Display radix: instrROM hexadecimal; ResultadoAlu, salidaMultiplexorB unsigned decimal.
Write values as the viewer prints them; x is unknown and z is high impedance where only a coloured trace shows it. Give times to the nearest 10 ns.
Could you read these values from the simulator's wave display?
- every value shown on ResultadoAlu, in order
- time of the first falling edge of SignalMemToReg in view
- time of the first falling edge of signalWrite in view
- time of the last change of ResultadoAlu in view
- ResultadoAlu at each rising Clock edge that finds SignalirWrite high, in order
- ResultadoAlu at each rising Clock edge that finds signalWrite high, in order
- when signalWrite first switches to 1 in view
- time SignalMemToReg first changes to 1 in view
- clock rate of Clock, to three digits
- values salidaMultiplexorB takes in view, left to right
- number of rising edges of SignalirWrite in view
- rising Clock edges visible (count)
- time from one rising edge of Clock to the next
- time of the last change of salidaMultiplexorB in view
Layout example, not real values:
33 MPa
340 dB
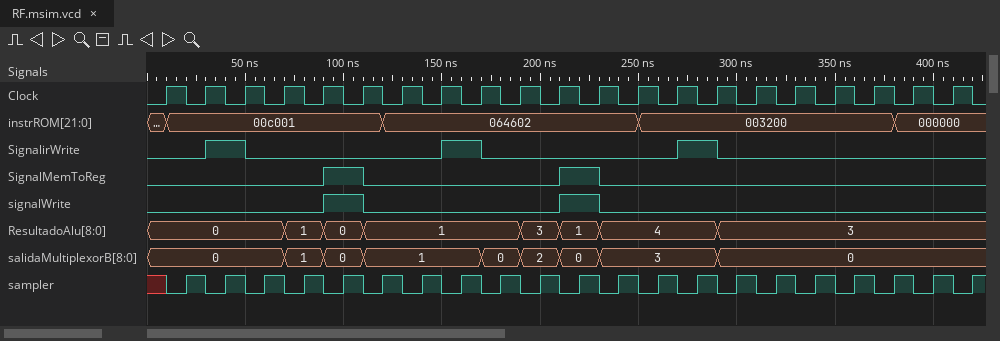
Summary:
0, 1, 0, 1, 3, 1, 4, 3
110 ns
110 ns
290 ns
0, 1, 4
0, 1
90 ns
90 ns
50.0 MHz
0, 1, 0, 1, 0, 2, 0, 3, 0
3
21
20 ns
290 ns
